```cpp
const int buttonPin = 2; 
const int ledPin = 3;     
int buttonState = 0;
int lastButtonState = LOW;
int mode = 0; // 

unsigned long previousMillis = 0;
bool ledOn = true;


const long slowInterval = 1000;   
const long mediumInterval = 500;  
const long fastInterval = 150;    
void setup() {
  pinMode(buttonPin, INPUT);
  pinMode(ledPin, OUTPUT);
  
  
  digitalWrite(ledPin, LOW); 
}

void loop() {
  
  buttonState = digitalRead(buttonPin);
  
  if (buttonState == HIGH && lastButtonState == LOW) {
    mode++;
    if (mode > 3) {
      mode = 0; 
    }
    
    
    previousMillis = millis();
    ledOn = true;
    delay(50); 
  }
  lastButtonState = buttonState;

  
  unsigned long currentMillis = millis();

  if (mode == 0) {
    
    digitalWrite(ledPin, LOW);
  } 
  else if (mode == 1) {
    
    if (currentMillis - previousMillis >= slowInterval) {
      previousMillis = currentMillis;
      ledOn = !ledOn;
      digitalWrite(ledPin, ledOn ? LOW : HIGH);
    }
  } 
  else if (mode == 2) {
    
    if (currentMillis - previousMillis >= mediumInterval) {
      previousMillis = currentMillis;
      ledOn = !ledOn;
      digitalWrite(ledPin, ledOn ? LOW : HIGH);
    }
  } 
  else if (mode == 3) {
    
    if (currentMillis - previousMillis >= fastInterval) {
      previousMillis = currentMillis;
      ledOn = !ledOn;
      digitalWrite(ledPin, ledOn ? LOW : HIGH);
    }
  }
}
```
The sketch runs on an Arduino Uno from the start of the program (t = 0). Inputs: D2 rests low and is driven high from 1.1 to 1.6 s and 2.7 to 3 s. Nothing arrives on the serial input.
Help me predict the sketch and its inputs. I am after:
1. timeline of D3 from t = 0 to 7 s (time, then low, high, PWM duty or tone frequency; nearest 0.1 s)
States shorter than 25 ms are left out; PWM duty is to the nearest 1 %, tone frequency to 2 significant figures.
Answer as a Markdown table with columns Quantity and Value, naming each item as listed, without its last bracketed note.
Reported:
| Quantity | Value |
|---|---|
| timeline of D3 from t = 0 to 7 s | 0 s low; 2.1 s high; 3.7 s low; 4.2 s high; 4.7 s low; 5.2 s high; 5.7 s low; 6.2 s high; 6.7 s low |
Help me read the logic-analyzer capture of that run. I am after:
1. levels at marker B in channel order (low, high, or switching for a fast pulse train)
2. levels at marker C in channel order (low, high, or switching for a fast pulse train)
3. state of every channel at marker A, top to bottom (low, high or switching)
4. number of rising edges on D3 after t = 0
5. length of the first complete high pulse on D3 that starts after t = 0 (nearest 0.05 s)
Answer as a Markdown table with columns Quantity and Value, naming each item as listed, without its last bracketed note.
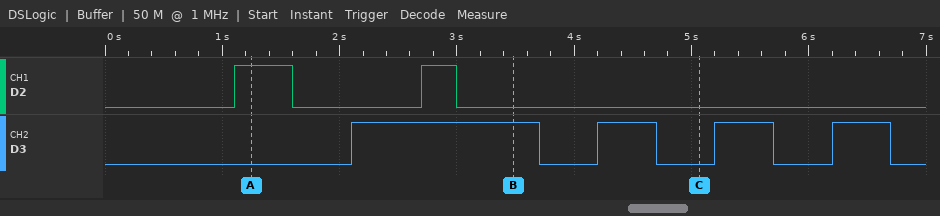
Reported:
| Quantity | Value |
|---|---|
| levels at marker B in channel order | D2 low, D3 high |
| levels at marker C in channel order | D2 low, D3 low |
| state of every channel at marker A, top to bottom | D2 high, D3 low |
| number of rising edges on D3 after t = 0 | 4 |
| length of the first complete high pulse on D3 that starts after t = 0 | 1.60 s |
